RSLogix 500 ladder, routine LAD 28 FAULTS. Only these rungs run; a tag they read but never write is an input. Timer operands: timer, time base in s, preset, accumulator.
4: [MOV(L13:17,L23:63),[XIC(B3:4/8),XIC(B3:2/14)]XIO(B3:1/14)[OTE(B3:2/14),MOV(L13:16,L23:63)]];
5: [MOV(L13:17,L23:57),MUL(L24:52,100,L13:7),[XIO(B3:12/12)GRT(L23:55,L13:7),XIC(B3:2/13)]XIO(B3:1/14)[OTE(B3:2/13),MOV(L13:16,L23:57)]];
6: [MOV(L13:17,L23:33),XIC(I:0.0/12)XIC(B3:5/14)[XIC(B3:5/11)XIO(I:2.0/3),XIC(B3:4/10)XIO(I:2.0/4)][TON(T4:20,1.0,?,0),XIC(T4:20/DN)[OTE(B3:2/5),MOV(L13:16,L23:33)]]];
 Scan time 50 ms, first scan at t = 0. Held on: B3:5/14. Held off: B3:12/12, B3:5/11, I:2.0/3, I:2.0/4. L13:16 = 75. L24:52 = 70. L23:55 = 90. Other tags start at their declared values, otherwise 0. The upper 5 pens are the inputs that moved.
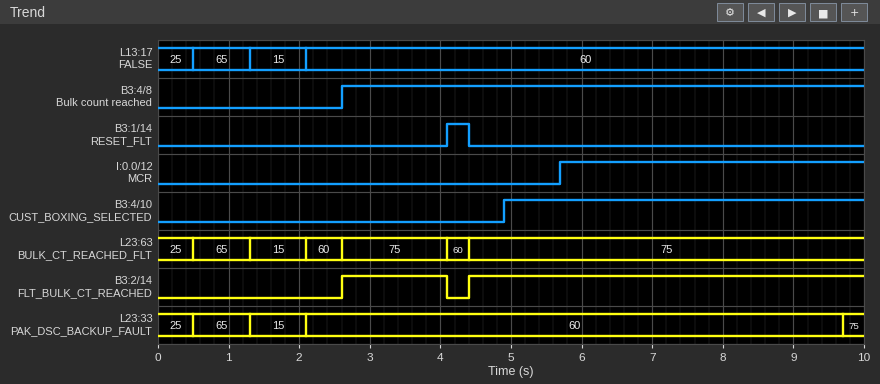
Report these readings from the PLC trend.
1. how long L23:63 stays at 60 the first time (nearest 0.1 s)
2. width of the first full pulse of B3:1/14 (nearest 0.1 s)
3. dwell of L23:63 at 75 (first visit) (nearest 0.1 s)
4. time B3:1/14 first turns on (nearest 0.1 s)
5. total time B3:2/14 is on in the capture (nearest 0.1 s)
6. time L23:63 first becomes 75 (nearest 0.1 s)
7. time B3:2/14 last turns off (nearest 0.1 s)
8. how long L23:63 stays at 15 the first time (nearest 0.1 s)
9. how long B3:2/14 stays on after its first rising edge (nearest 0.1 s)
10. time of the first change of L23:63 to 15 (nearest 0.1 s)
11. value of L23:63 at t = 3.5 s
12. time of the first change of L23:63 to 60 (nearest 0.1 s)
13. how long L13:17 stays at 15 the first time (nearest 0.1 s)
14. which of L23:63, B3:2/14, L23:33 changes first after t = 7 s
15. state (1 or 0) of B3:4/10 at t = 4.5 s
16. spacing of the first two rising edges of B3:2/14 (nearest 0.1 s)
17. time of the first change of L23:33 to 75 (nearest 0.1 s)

0.5 s
0.3 s
1.5 s
4.1 s
7.1 s
2.6 s
4.1 s
0.8 s
1.5 s
1.3 s
75
2.1 s
0.8 s
L23:33
0
1.8 s
9.7 s
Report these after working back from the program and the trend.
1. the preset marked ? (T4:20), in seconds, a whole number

4 s
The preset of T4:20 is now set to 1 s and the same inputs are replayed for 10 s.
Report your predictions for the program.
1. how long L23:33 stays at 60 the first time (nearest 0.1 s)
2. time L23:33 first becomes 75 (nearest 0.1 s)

4.6 s
6.7 s
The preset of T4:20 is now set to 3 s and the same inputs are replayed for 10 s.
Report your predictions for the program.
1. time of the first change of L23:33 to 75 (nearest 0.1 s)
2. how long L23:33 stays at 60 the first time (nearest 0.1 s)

8.7 s
6.6 s
